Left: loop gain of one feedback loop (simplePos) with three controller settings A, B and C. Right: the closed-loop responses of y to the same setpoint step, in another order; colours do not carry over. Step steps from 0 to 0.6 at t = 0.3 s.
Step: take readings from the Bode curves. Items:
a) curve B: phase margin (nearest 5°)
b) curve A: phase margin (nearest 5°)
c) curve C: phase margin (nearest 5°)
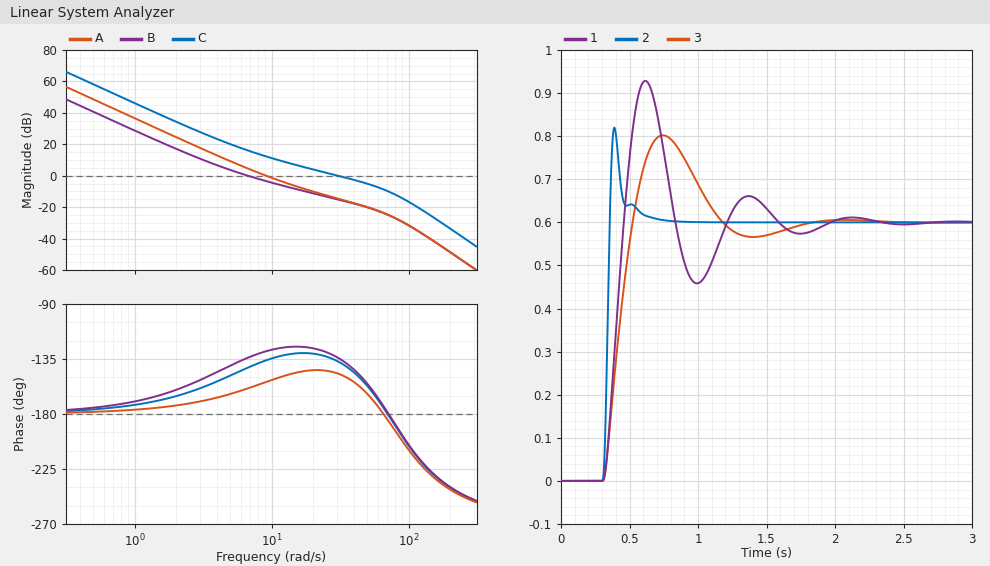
45°
25°
45°
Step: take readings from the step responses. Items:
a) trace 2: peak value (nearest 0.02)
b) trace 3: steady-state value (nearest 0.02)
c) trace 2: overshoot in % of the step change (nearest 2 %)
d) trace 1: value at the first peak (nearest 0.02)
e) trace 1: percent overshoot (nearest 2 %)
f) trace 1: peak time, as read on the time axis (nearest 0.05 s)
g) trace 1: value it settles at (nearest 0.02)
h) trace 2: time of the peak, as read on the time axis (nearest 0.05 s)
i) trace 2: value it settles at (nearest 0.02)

0.82
0.60
36 %
0.92
54 %
0.60 s
0.60
0.40 s
0.60
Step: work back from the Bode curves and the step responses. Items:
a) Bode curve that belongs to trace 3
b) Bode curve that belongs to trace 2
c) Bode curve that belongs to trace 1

B
C
A
